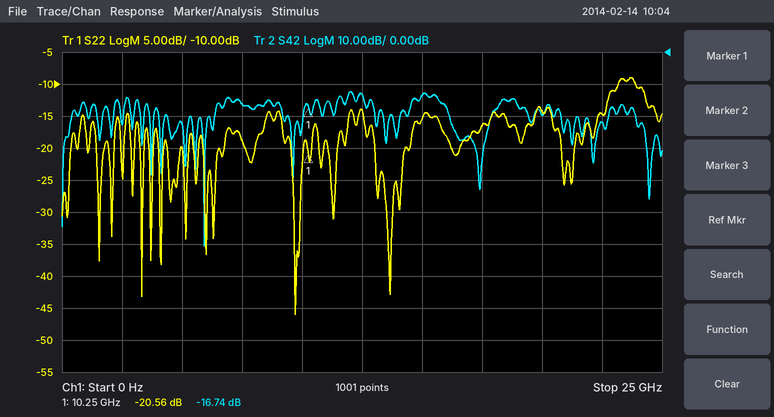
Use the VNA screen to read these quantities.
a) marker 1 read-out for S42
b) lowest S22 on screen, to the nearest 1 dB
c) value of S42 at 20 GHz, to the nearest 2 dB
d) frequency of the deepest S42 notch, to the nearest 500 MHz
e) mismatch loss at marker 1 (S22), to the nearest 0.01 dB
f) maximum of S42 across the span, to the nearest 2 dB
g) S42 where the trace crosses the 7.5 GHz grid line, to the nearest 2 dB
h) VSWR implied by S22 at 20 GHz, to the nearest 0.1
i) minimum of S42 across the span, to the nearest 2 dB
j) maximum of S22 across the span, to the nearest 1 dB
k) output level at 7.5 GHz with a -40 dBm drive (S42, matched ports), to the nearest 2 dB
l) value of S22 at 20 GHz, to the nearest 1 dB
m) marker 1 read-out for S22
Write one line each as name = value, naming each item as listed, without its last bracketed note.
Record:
marker 1 read-out for S42 = -16.74 dB
lowest S22 on screen, to the nearest 1 dB = -46 dB
value of S42 at 20 GHz, to the nearest 2 dB = -20 dB
frequency of the deepest S42 notch, to the nearest 500 MHz = 6.0 GHz
mismatch loss at marker 1 (S22), to the nearest 0.01 dB = 0.04 dB
maximum of S42 across the span, to the nearest 2 dB = -12 dB
S42 where the trace crosses the 7.5 GHz grid line, to the nearest 2 dB = -16 dB
VSWR implied by S22 at 20 GHz, to the nearest 0.1 = 1.5
minimum of S42 across the span, to the nearest 2 dB = -60 dB
maximum of S22 across the span, to the nearest 1 dB = -9 dB
output level at 7.5 GHz with a -40 dBm drive (S42, matched ports), to the nearest 2 dB = -56 dBm
value of S22 at 20 GHz, to the nearest 1 dB = -14 dB
marker 1 read-out for S22 = -20.56 dB
